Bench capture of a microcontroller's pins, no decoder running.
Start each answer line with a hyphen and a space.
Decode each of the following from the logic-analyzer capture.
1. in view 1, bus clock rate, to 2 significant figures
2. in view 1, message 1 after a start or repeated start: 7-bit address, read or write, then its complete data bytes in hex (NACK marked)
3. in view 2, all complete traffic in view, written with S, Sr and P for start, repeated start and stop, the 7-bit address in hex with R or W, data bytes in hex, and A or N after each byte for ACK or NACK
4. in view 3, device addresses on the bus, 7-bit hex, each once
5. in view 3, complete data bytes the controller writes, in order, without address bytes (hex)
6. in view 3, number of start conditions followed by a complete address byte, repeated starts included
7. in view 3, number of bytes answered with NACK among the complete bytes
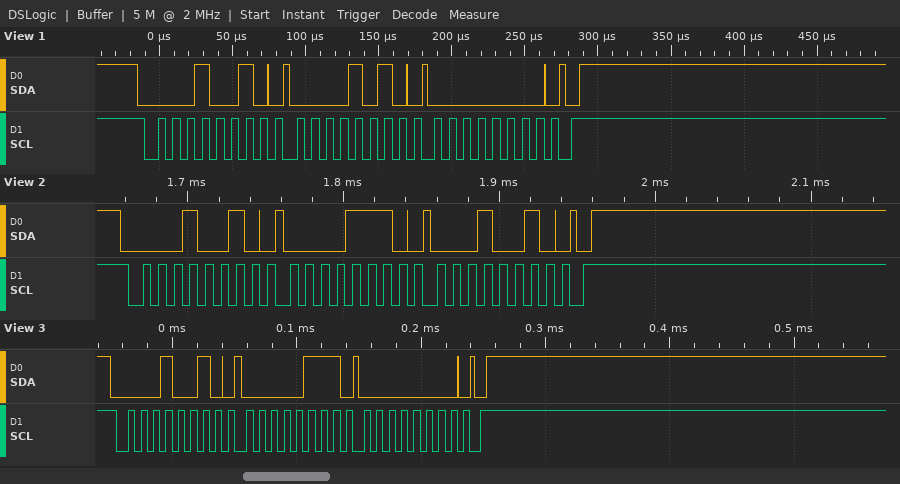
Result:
- 100 kHz
- 0x09 write: 0A 00
- S 09W A 0E A 12 A P
- 0x09
- 07 00
- 1
- 0
